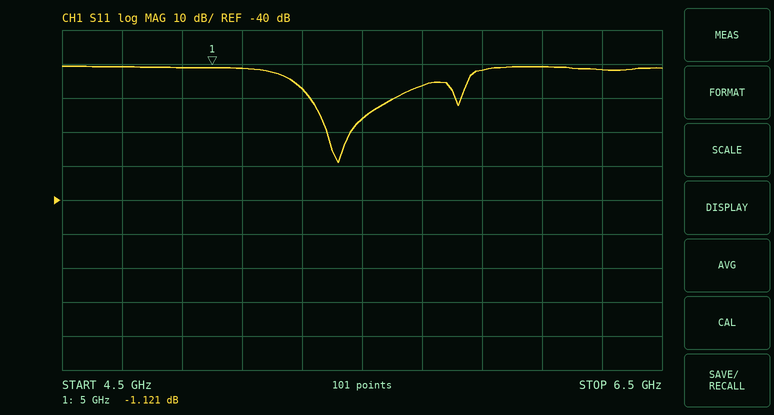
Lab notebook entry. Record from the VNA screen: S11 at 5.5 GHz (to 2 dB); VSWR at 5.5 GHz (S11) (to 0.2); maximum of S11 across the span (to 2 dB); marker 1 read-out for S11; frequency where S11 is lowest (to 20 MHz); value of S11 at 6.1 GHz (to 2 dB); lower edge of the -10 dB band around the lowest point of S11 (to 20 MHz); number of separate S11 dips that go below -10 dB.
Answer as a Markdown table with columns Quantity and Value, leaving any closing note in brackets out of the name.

| Quantity | Value |
|---|---|
| S11 at 5.5 GHz | -16 dB |
| VSWR at 5.5 GHz (S11) | 1.4 |
| maximum of S11 across the span | 0 dB |
| marker 1 read-out for S11 | -1.121 dB |
| frequency where S11 is lowest | 5.42 GHz |
| value of S11 at 6.1 GHz | 0 dB |
| lower edge of the -10 dB band around the lowest point of S11 | 5.32 GHz |
| number of separate S11 dips that go below -10 dB | 2 |
